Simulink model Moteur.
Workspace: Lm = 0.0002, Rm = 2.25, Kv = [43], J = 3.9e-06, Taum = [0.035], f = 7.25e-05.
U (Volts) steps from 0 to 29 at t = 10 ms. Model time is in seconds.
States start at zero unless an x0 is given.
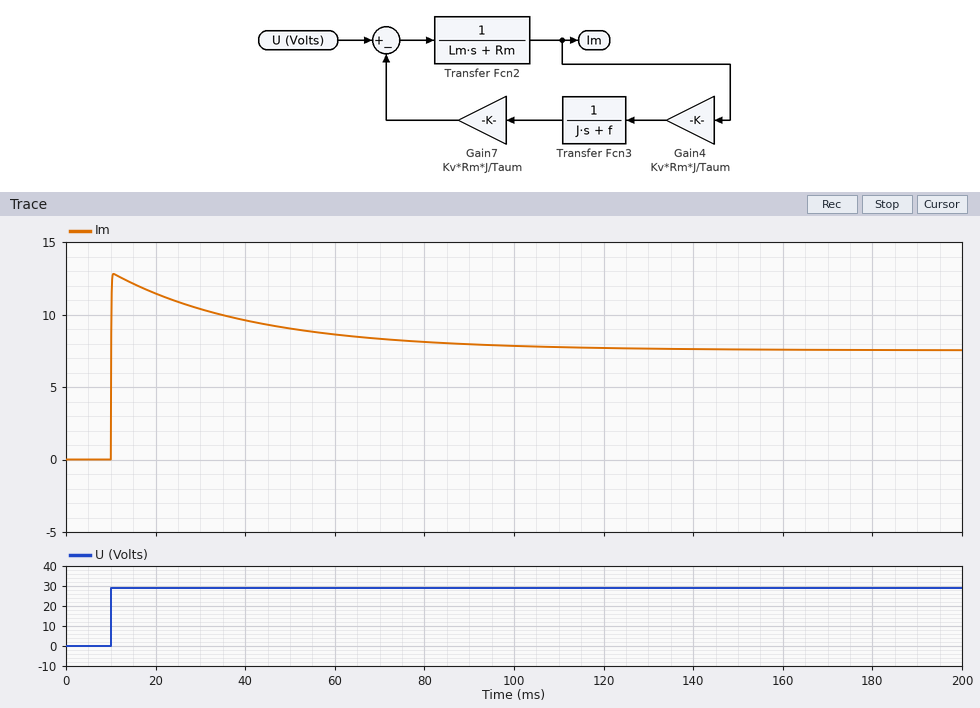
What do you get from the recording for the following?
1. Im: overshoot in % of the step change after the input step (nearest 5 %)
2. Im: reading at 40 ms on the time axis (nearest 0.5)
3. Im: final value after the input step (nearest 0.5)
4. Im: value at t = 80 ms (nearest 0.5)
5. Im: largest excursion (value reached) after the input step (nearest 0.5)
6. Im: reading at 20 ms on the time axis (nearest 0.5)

70 %
9.5
7.5
8.0
13.0
11.5
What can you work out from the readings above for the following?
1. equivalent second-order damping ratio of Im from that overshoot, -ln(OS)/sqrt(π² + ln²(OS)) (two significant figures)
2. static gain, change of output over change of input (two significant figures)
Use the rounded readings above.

0.11
0.26
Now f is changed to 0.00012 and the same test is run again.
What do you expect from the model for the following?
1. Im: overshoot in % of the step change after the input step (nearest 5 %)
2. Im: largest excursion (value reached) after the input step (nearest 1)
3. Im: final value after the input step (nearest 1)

40 %
13
9
